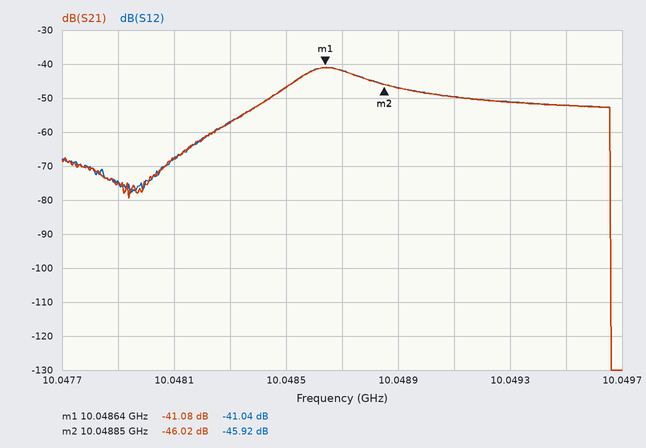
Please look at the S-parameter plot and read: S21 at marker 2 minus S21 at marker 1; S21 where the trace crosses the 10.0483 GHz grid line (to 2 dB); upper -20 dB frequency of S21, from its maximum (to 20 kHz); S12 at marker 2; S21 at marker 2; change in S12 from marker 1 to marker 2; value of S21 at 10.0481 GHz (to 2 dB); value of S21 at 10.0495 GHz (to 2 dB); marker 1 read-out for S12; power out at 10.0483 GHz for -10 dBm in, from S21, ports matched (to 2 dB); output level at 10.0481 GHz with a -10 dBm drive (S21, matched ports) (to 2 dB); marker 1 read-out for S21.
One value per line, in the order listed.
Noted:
-4.94 dB
-58 dB
10.04966 GHz
-45.92 dB
-46.02 dB
-4.88 dB
-68 dB
-52 dB
-41.04 dB
-68 dBm
-78 dBm
-41.08 dB
